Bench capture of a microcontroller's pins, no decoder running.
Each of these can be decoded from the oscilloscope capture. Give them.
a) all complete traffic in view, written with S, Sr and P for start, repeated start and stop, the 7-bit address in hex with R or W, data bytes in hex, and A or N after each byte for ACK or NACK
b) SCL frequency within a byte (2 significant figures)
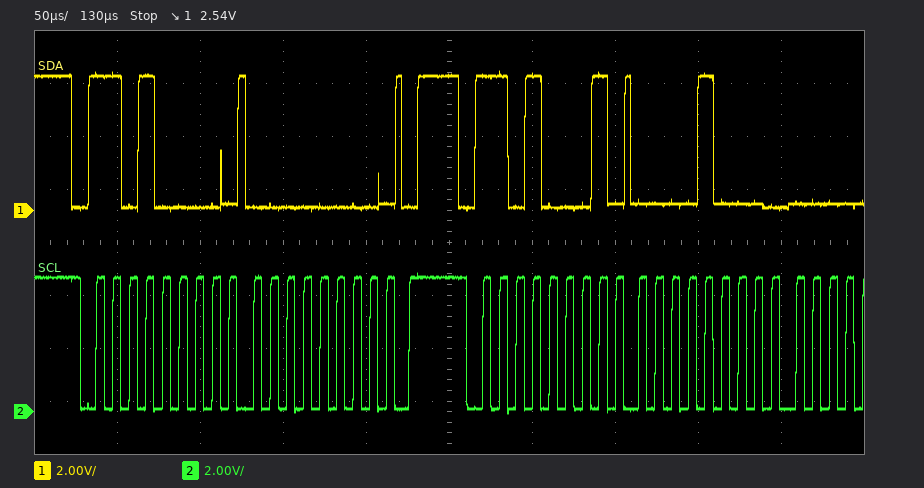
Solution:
S 68W A 00 A P S 68R A 08 A
100 kHz
